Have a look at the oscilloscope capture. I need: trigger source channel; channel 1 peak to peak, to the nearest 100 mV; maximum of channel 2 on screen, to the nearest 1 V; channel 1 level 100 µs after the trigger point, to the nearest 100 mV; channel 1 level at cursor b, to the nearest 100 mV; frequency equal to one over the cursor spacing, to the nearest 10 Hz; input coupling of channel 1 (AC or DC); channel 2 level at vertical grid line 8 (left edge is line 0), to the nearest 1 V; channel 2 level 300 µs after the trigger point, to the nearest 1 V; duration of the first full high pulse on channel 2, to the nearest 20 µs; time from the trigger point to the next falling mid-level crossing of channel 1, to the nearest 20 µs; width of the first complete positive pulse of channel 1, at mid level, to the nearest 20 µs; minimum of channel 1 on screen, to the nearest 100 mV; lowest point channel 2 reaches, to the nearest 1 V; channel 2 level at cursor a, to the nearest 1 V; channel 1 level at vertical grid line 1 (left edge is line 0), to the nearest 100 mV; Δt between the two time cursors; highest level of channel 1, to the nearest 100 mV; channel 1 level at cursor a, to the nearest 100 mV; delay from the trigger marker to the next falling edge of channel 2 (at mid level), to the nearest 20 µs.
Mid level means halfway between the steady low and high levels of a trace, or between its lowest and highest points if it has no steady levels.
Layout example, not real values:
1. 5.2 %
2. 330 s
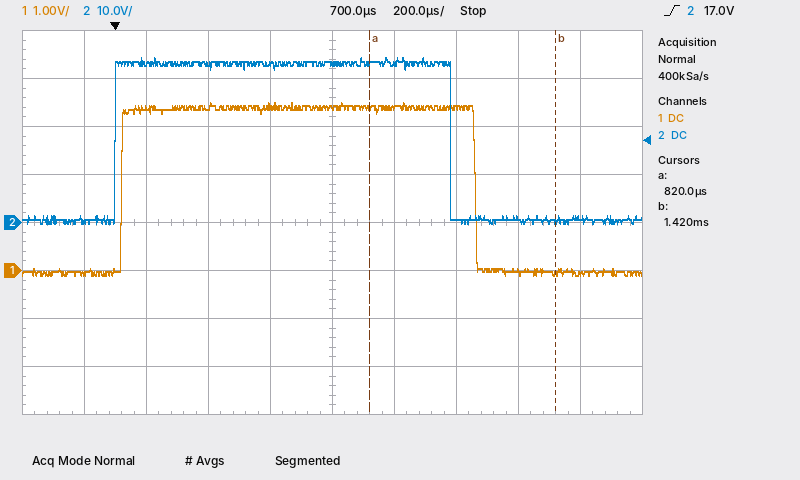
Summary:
1. channel 2
2. 3.6 V
3. 34 V
4. 3.4 V
5. 0.0 V
6. 1.67 kHz
7. DC
8. 1 V
9. 33 V
10. 1.08 ms
11. 1.16 ms
12. 1.14 ms
13. -100 mV
14. 0 V
15. 33 V
16. -100 mV
17. 600 µs
18. 3.5 V
19. 3.4 V
20. 1.08 ms
